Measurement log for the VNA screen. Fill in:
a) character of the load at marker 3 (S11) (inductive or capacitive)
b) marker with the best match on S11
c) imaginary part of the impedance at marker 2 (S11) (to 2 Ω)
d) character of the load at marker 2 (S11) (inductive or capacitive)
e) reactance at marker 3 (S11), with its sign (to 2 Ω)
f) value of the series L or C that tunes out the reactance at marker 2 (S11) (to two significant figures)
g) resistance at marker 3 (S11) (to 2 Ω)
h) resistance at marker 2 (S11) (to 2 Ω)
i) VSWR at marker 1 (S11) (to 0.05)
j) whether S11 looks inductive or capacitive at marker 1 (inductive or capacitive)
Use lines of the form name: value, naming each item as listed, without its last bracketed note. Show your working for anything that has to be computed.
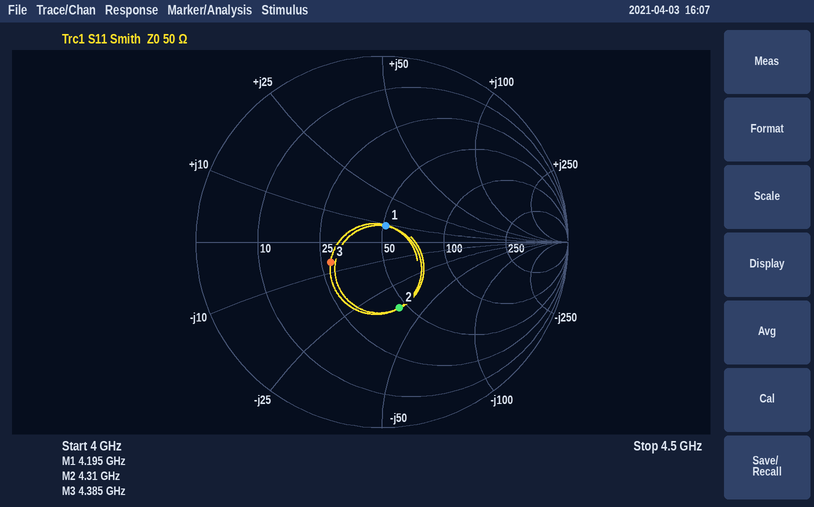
character of the load at marker 3 (S11): capacitive
marker with the best match on S11: marker 1
imaginary part of the impedance at marker 2 (S11): -38 Ω
character of the load at marker 2 (S11): capacitive
reactance at marker 3 (S11), with its sign: -6 Ω
value of the series L or C that tunes out the reactance at marker 2 (S11): L = 38 Ω/(2π × 4.31 GHz) ≈ 1.4 nH
resistance at marker 3 (S11): 28 Ω
resistance at marker 2 (S11): 46 Ω
VSWR at marker 1 (S11): 1.20
whether S11 looks inductive or capacitive at marker 1: inductive
